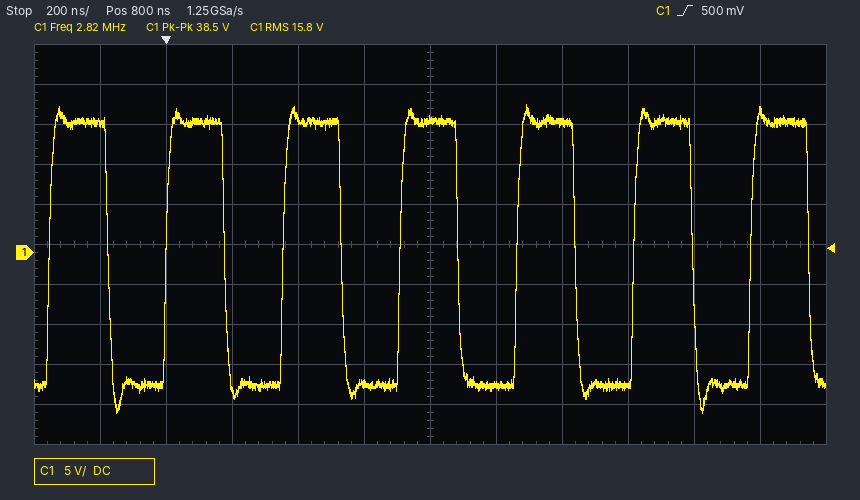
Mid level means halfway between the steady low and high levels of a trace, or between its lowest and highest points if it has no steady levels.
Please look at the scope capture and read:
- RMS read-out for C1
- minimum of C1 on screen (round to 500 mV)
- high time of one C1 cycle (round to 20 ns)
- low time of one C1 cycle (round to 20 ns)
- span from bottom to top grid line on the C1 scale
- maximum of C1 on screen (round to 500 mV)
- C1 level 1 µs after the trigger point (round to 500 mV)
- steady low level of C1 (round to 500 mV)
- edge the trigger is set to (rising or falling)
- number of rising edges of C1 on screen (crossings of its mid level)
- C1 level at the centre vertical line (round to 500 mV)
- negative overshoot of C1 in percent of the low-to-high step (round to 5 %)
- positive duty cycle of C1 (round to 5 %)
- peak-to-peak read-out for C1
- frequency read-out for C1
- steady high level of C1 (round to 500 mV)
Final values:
15.8 V
-20.0 V
180 ns
180 ns
50 V
18.5 V
-16.5 V
-16.5 V
rising
7
16.5 V
10 %
50 %
38.5 V
2.82 MHz
16.5 V
